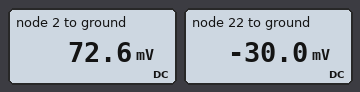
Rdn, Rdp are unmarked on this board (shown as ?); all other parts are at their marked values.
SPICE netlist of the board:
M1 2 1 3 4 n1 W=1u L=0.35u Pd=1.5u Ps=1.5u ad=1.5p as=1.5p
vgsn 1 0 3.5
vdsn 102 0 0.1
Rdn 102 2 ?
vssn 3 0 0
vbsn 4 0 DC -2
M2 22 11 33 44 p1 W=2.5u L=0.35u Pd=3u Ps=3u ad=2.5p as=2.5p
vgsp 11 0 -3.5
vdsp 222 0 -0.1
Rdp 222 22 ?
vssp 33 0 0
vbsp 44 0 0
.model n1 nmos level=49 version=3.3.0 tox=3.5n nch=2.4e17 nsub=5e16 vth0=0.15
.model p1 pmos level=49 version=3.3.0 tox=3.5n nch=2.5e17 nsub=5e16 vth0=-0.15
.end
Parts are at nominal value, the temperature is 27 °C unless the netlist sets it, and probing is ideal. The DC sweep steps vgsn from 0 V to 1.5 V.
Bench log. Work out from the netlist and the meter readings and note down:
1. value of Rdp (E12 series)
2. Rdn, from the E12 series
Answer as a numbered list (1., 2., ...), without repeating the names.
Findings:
1. 1.8 kΩ
2. 330 Ω
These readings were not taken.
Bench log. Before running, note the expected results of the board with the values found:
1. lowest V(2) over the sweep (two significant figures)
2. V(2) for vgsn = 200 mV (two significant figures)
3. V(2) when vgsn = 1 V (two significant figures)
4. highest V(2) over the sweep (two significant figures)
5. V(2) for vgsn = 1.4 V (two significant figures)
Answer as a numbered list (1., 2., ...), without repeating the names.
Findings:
1. 84 mV
2. 100 mV
3. 92 mV
4. 100 mV
5. 85 mV
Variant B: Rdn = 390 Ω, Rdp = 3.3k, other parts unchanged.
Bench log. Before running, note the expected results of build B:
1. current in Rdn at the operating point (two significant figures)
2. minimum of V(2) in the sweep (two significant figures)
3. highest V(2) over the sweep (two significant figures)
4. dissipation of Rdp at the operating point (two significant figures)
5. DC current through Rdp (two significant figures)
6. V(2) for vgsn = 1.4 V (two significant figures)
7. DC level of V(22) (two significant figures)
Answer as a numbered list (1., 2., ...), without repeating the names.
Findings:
1. 79 µA
2. 82 mV
3. 100 mV
4. 2.0 µW
5. 25 µA
6. 83 mV
7. -19 mV
